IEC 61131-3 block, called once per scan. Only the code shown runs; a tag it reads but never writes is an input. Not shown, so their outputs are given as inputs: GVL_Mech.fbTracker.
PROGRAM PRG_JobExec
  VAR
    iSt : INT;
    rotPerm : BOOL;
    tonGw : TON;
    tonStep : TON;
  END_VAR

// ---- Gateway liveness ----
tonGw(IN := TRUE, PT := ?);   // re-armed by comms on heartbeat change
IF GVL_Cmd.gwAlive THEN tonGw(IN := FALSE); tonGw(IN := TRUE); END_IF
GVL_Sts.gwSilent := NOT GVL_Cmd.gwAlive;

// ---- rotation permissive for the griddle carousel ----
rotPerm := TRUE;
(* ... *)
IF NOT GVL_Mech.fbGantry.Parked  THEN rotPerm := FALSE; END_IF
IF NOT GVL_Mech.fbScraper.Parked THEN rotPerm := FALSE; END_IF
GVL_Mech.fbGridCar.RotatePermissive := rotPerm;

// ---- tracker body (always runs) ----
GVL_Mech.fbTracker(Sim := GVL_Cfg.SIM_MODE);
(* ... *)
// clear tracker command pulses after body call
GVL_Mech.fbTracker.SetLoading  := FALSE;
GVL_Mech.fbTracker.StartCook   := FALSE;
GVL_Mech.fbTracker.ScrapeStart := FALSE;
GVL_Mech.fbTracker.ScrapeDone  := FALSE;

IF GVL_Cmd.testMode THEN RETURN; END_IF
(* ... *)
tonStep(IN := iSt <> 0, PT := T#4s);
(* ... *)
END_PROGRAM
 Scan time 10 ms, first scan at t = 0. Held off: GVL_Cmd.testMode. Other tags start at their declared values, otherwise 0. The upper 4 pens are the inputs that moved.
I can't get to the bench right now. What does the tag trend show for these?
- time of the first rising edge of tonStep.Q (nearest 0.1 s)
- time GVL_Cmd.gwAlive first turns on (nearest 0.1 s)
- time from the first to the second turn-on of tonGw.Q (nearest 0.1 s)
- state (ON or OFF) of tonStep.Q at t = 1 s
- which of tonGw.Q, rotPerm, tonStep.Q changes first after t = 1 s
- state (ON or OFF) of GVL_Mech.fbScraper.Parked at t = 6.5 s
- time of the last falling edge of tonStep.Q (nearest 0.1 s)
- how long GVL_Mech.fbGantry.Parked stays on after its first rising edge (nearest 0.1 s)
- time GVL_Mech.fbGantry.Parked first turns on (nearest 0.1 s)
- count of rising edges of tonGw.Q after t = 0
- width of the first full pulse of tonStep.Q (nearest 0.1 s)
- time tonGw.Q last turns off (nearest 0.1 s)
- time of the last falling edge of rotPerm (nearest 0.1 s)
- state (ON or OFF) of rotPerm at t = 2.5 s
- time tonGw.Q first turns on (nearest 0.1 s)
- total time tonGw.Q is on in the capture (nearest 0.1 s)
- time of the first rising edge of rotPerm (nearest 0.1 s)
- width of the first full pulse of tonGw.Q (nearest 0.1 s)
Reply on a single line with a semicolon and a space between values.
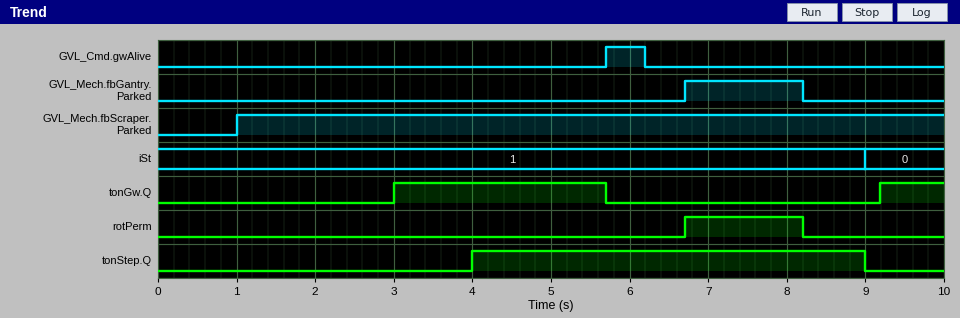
4.0 s; 5.7 s; 6.2 s; OFF; tonGw.Q; ON; 9.0 s; 1.5 s; 6.7 s; 2; 5.0 s; 5.7 s; 8.2 s; OFF; 3.0 s; 3.5 s; 6.7 s; 2.7 s
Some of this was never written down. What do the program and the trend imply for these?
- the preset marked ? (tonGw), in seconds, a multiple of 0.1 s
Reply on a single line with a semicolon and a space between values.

3.0 s
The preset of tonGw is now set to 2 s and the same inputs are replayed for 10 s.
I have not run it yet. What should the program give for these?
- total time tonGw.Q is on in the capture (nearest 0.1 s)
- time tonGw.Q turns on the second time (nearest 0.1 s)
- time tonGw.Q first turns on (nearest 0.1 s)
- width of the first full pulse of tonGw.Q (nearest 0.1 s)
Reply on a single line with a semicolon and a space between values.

5.5 s; 8.2 s; 2.0 s; 3.7 s
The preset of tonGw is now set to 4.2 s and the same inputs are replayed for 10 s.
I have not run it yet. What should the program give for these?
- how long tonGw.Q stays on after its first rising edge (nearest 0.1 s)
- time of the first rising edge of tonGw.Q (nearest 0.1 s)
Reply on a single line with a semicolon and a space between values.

1.5 s; 4.2 s
